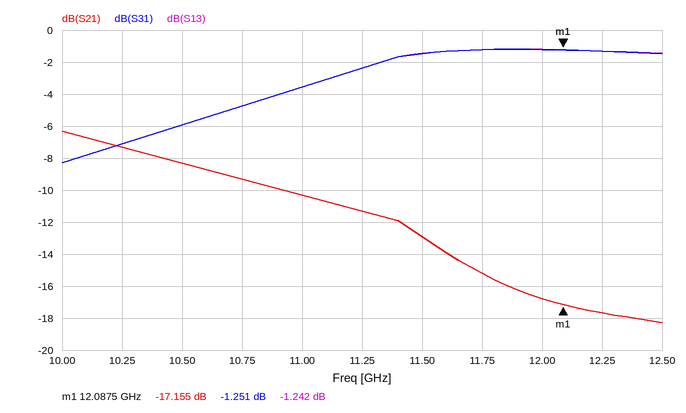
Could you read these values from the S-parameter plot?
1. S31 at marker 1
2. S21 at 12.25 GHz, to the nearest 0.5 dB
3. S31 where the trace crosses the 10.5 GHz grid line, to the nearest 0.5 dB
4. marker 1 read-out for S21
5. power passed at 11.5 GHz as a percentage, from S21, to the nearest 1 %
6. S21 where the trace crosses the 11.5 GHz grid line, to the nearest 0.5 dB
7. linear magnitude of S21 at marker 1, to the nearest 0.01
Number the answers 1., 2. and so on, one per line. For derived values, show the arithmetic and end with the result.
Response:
1. -1.251 dB
2. -17.5 dB
3. -6.0 dB
4. -17.155 dB
5. 10^(-13/10) ≈ 5 %
6. -13.0 dB
7. 10^(-17.155/20) ≈ 0.14
